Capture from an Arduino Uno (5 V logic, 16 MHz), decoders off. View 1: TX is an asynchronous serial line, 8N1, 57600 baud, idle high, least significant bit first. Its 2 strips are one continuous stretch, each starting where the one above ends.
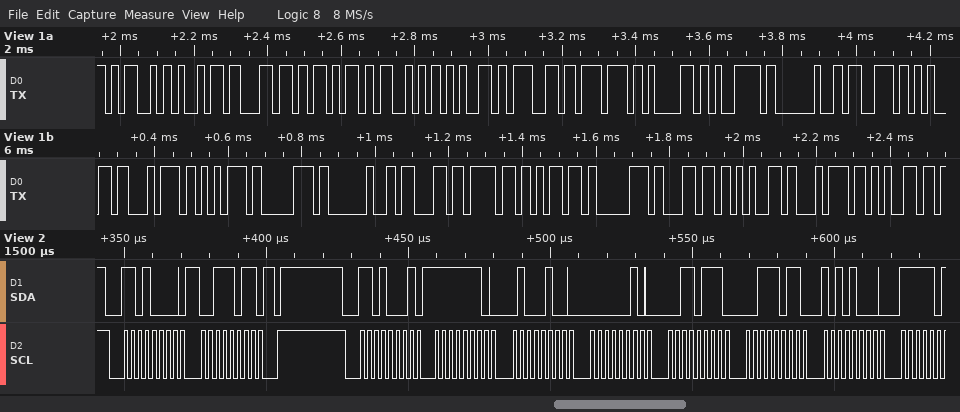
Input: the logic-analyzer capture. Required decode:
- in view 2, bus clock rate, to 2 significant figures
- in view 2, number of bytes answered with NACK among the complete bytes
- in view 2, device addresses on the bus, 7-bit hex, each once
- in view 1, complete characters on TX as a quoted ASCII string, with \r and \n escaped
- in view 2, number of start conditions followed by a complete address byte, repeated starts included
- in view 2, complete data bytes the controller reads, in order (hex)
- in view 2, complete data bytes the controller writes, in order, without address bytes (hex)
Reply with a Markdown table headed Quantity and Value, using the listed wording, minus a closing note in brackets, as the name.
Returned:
| Quantity | Value |
|---|---|
| in view 2, bus clock rate, to 2 significant figures | 400 kHz |
| in view 2, number of bytes answered with NACK among the complete bytes | 0 |
| in view 2, device addresses on the bus, 7-bit hex, each once | 0x68 |
| in view 1, complete characters on TX as a quoted ASCII string, with \r and \n escaped | "MilkSegway setup complete" |
| in view 2, number of start conditions followed by a complete address byte, repeated starts included | 2 |
| in view 2, complete data bytes the controller reads, in order | FE 44 02 37 3B A8 |
| in view 2, complete data bytes the controller writes, in order, without address bytes | 3B |
